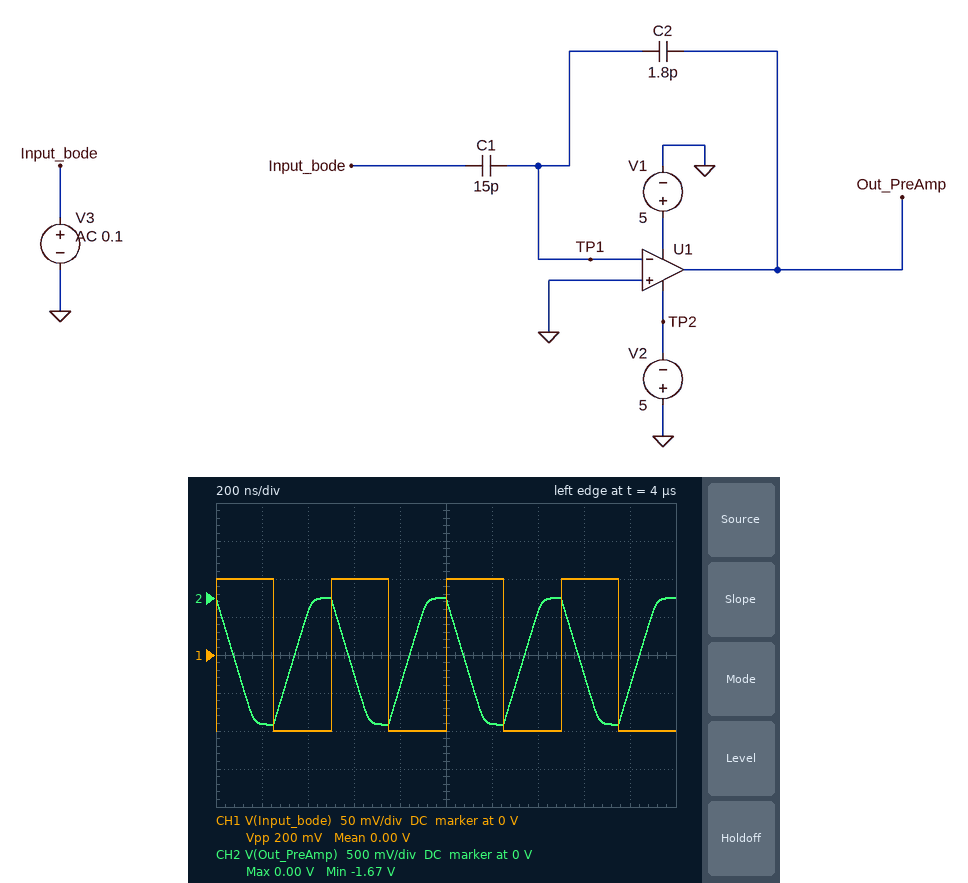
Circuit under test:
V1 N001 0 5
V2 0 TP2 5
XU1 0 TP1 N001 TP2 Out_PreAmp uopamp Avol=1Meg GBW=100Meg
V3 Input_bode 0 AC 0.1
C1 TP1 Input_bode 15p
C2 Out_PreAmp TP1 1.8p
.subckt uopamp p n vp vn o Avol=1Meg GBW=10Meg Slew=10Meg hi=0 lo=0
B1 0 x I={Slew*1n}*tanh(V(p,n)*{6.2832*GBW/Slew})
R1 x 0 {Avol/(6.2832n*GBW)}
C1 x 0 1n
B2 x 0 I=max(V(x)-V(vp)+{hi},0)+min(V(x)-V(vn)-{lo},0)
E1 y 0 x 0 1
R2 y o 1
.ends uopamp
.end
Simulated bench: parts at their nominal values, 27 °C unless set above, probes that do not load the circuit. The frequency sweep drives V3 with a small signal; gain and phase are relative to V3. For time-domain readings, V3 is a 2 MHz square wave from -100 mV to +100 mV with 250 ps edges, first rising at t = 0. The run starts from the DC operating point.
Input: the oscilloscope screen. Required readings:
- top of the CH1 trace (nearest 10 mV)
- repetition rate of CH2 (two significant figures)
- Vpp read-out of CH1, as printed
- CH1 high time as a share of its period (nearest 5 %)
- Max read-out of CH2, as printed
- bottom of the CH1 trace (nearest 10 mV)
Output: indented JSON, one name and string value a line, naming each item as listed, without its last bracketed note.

{
  "top of the CH1 trace": "100 mV",
  "repetition rate of CH2": "2.0 MHz",
  "Vpp read-out of CH1, as printed": "200 mV",
  "CH1 high time as a share of its period": "50 %",
  "Max read-out of CH2, as printed": "0.00 V",
  "bottom of the CH1 trace": "-100 mV"
}
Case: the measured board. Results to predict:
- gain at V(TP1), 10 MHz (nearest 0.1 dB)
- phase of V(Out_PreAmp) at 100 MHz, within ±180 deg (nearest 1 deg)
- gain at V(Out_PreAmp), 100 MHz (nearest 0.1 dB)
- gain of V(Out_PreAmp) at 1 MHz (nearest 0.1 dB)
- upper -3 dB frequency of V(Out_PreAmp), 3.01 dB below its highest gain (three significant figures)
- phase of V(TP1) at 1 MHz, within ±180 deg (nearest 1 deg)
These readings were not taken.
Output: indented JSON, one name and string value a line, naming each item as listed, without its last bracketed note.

{
  "gain at V(TP1), 10 MHz": "-4.3 dB",
  "phase of V(Out_PreAmp) at 100 MHz, within ±180 deg": "96 deg",
  "gain at V(Out_PreAmp), 100 MHz": "-1.0 dB",
  "gain of V(Out_PreAmp) at 1 MHz": "18.4 dB",
  "upper -3 dB frequency of V(Out_PreAmp), 3.01 dB below its highest gain": "10.7 MHz",
  "phase of V(TP1) at 1 MHz, within ±180 deg": "85 deg"
}
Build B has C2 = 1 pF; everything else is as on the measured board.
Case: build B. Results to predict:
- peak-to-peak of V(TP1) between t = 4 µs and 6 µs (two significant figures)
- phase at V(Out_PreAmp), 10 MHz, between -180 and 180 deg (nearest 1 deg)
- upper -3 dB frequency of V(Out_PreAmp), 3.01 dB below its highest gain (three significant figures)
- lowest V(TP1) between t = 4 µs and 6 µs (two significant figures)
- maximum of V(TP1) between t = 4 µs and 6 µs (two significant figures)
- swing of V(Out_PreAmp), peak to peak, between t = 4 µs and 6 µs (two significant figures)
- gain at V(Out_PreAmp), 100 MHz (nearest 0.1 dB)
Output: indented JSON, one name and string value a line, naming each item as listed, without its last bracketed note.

{
  "peak-to-peak of V(TP1) between t = 4 µs and 6 µs": "340 mV",
  "phase at V(Out_PreAmp), 10 MHz, between -180 and 180 deg": "122 deg",
  "upper -3 dB frequency of V(Out_PreAmp), 3.01 dB below its highest gain": "6.25 MHz",
  "lowest V(TP1) between t = 4 µs and 6 µs": "-170 mV",
  "maximum of V(TP1) between t = 4 µs and 6 µs": "170 mV",
  "swing of V(Out_PreAmp), peak to peak, between t = 4 µs and 6 µs": "2.5 V",
  "gain at V(Out_PreAmp), 100 MHz": "-0.6 dB"
}
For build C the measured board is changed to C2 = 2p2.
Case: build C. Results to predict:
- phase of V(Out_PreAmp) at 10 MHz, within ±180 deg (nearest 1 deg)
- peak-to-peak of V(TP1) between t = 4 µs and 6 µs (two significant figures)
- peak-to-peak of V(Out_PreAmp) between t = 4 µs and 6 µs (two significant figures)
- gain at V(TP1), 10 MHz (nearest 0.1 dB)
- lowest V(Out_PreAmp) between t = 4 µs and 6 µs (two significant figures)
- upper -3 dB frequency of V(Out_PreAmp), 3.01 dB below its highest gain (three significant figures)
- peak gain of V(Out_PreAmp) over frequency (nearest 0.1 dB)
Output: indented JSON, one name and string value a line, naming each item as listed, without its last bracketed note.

{
  "phase of V(Out_PreAmp) at 10 MHz, within ±180 deg": "142 deg",
  "peak-to-peak of V(TP1) between t = 4 µs and 6 µs": "350 mV",
  "peak-to-peak of V(Out_PreAmp) between t = 4 µs and 6 µs": "1.4 V",
  "gain at V(TP1), 10 MHz": "-5.4 dB",
  "lowest V(Out_PreAmp) between t = 4 µs and 6 µs": "-1.4 V",
  "upper -3 dB frequency of V(Out_PreAmp), 3.01 dB below its highest gain": "12.8 MHz",
  "peak gain of V(Out_PreAmp) over frequency": "16.7 dB"
}
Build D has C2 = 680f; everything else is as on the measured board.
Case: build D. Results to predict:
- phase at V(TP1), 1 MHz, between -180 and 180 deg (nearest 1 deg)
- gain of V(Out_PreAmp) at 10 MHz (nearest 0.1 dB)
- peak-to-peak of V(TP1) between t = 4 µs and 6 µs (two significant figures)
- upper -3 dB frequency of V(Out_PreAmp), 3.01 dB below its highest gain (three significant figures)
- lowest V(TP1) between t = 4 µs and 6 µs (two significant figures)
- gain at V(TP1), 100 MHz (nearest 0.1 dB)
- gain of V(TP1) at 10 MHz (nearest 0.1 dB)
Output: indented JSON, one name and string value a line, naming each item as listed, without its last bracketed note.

{
  "phase at V(TP1), 1 MHz, between -180 and 180 deg": "77 deg",
  "gain of V(Out_PreAmp) at 10 MHz": "18.9 dB",
  "peak-to-peak of V(TP1) between t = 4 µs and 6 µs": "300 mV",
  "upper -3 dB frequency of V(Out_PreAmp), 3.01 dB below its highest gain": "4.34 MHz",
  "lowest V(TP1) between t = 4 µs and 6 µs": "-130 mV",
  "gain at V(TP1), 100 MHz": "-0.4 dB",
  "gain of V(TP1) at 10 MHz": "-1.1 dB"
}
